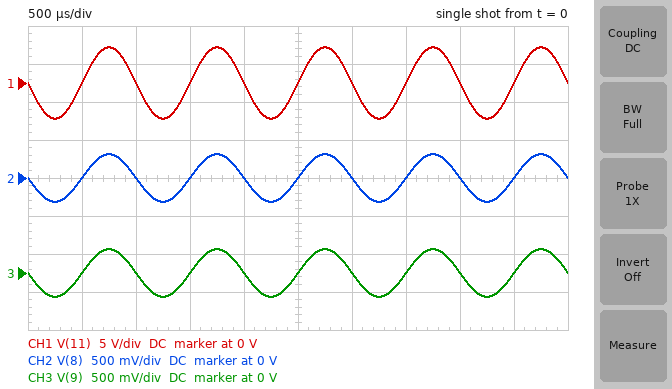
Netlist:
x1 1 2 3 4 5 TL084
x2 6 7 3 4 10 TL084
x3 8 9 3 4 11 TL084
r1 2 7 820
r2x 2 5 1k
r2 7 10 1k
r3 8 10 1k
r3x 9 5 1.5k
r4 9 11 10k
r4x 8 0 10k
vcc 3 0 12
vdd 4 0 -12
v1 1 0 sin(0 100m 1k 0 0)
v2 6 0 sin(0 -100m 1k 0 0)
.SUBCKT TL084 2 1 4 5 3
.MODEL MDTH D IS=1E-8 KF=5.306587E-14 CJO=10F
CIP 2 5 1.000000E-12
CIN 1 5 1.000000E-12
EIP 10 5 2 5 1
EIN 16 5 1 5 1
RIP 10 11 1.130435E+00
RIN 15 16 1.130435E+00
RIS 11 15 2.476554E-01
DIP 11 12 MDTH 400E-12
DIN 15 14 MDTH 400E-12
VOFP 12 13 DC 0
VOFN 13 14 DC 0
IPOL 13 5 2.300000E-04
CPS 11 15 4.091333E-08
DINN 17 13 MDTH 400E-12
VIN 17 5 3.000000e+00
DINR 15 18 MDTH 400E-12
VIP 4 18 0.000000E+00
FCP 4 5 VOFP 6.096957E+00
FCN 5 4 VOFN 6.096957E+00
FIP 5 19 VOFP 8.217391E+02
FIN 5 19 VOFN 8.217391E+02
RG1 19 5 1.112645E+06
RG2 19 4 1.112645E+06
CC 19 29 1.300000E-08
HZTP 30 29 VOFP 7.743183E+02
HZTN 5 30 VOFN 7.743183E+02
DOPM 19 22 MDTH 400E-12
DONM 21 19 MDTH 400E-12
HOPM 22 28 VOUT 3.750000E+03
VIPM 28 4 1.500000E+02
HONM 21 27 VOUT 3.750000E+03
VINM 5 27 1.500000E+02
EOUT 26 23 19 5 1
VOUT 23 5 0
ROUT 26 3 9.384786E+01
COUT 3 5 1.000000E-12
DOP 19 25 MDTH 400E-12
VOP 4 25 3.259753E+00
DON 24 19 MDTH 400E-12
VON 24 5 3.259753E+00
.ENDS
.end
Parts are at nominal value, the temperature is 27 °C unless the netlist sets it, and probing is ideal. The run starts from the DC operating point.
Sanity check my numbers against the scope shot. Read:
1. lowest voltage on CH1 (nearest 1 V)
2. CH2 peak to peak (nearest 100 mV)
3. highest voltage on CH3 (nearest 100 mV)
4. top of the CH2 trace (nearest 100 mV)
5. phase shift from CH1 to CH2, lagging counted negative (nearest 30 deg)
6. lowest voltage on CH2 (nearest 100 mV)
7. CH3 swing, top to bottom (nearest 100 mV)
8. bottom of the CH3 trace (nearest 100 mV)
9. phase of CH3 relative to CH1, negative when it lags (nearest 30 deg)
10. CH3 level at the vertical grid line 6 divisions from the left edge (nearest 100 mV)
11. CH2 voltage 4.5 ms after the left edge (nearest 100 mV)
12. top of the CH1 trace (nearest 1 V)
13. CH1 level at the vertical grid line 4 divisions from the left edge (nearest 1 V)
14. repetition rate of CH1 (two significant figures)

-5 V
600 mV
300 mV
300 mV
0 deg
-300 mV
600 mV
-300 mV
0 deg
0 V
0 V
5 V
0 V
1.0 kHz
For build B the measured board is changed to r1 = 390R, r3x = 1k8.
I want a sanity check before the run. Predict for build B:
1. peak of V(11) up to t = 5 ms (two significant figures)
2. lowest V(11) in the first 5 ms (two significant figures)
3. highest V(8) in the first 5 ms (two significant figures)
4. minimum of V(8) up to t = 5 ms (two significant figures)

7.1 V
-7.1 V
560 mV
-560 mV
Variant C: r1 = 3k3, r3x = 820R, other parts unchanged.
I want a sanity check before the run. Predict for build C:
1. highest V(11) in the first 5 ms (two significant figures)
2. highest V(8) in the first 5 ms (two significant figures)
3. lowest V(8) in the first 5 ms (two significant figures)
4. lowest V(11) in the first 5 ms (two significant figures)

3.9 V
150 mV
-150 mV
-3.9 V
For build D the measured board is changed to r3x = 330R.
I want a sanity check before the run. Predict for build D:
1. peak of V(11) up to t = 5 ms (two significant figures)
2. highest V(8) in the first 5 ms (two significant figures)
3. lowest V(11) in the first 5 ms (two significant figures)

9.6 V
310 mV
-9.6 V
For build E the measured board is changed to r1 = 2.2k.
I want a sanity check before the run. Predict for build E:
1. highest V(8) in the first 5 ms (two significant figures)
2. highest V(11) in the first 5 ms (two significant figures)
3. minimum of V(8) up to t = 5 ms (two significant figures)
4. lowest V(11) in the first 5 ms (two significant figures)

170 mV
2.6 V
-170 mV
-2.6 V
